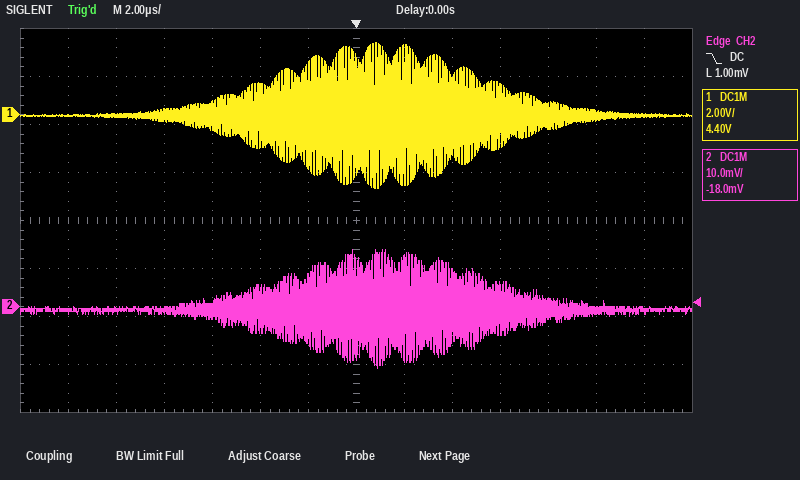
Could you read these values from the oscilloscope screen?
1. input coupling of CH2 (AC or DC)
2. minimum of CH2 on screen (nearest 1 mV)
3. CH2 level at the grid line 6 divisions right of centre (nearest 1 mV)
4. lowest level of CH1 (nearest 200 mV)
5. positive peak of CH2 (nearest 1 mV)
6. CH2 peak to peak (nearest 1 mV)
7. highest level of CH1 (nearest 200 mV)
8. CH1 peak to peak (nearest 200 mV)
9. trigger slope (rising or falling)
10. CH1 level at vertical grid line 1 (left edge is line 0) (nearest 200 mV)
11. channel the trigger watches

DC
-13 mV
-1 mV
-3.0 V
12 mV
25 mV
3.0 V
6.0 V
falling
0.0 V
CH2
